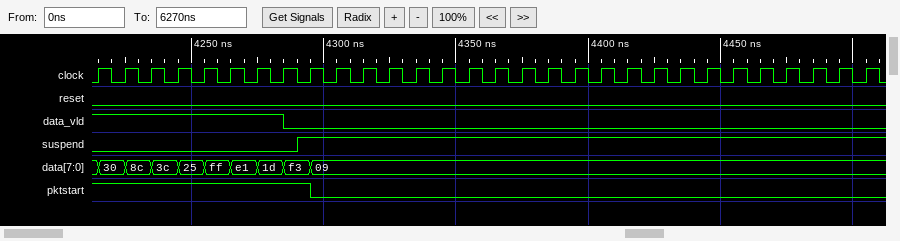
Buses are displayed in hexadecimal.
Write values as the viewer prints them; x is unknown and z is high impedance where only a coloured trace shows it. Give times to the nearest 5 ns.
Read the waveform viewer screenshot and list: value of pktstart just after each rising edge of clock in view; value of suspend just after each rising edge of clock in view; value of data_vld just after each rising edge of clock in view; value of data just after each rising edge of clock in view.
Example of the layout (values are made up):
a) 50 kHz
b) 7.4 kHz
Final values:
a) 1 1 1 1 1 1 1 1 0 0 0 0 0 0 0 0 0 0 0 0 0 0 0 0 0 0 0 0 0 0
b) 0 0 0 0 0 0 0 0 1 1 1 1 1 1 1 1 1 1 1 1 1 1 1 1 1 1 1 1 1 1
c) 1 1 1 1 1 1 1 0 0 0 0 0 0 0 0 0 0 0 0 0 0 0 0 0 0 0 0 0 0 0
d) 30, 8c, 3c, 25, ff, e1, 1d, f3, 09, 09, 09, 09, 09, 09, 09, 09, 09, 09, 09, 09, 09, 09, 09, 09, 09, 09, 09, 09, 09, 09
